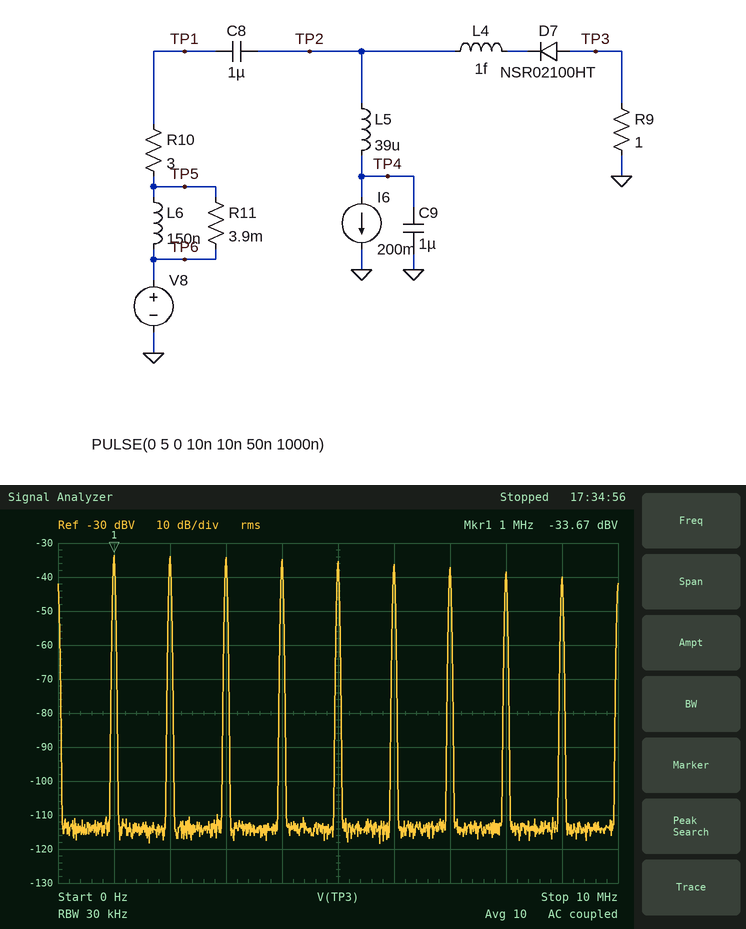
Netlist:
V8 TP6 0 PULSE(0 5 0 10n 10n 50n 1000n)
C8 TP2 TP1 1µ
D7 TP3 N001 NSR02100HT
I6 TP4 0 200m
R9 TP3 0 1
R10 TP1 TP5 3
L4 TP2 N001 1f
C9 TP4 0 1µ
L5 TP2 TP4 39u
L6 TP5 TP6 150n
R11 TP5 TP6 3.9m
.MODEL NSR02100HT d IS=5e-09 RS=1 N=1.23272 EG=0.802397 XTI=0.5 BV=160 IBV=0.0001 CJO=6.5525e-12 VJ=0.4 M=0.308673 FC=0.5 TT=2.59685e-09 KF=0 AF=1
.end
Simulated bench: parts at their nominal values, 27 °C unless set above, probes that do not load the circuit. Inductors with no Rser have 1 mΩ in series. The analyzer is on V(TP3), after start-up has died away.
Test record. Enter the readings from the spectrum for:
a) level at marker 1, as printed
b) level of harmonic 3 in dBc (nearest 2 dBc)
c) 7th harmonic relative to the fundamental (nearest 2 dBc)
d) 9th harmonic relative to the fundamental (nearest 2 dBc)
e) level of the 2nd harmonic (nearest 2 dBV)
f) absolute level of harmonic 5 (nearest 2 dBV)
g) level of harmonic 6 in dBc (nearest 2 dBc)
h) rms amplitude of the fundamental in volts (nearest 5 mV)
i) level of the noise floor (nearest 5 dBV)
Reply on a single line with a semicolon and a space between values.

-33.67 dBV; 0 dBc; -4 dBc; -6 dBc; -34 dBV; -36 dBV; -2 dBc; 20 mV; -115 dBV
